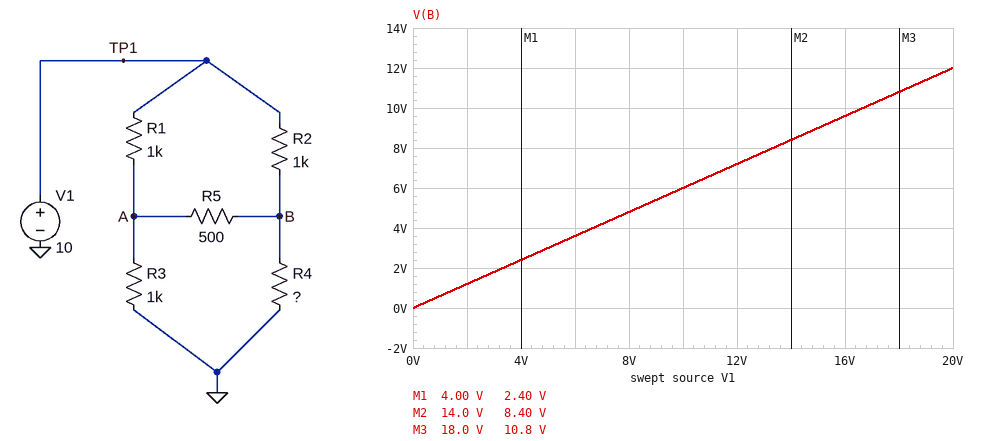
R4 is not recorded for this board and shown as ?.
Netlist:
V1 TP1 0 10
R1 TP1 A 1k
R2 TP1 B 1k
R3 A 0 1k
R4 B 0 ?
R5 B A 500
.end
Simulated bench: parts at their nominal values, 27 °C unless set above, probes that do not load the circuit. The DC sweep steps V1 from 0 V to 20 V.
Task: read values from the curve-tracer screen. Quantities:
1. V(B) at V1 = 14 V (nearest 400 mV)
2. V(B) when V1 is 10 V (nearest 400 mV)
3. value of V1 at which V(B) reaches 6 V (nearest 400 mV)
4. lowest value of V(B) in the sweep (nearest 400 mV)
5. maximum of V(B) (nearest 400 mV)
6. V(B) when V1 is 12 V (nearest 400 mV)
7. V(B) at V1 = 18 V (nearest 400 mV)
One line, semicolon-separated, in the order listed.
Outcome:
8.4 V; 6.0 V; 10.0 V; 0 V; 12.0 V; 7.2 V; 10.8 V
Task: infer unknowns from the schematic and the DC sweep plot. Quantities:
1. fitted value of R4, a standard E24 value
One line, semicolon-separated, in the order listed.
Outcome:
2 kΩ
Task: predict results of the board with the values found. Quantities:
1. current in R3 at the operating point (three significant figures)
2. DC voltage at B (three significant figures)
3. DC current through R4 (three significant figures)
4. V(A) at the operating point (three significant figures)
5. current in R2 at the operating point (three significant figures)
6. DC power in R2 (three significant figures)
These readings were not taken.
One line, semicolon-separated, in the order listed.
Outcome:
5.50 mA; 6.00 V; 3.00 mA; 5.50 V; 4.00 mA; 16.0 mW
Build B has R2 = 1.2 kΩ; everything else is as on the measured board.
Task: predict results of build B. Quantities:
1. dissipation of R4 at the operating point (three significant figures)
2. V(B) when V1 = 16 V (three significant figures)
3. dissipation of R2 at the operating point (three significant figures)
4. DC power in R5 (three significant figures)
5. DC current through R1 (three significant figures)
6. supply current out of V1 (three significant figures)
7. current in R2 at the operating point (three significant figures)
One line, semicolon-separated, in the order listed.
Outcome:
16.3 mW; 9.14 V; 15.3 mW; 255 µW; 4.64 mA; 8.21 mA; 3.57 mA
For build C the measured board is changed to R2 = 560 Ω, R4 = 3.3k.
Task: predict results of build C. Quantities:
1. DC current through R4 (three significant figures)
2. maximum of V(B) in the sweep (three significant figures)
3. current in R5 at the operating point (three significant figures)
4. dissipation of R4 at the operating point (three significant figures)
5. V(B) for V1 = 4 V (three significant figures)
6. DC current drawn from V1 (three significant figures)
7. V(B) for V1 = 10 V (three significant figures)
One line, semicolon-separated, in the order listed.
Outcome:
2.24 mA; 14.8 V; 2.40 mA; 16.6 mW; 2.96 V; 8.44 mA; 7.40 V
